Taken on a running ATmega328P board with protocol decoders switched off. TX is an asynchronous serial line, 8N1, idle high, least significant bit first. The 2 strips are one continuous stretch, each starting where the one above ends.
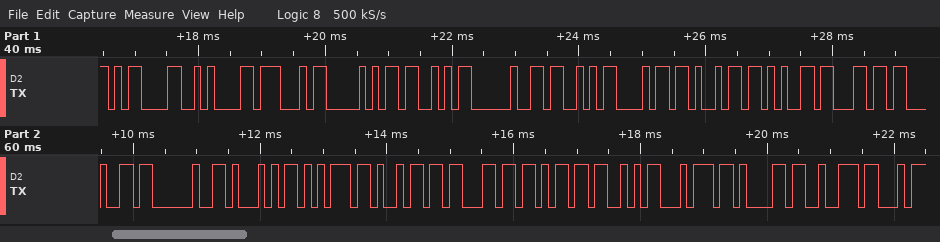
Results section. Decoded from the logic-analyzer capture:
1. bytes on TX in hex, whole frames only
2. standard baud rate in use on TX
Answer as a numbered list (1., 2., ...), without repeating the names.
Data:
1. 0D 0A 47 50 53 20 53 68 69 65 6C 64 20 51 75 69 63 6B 53 74 61 72
2. 9600 baud
